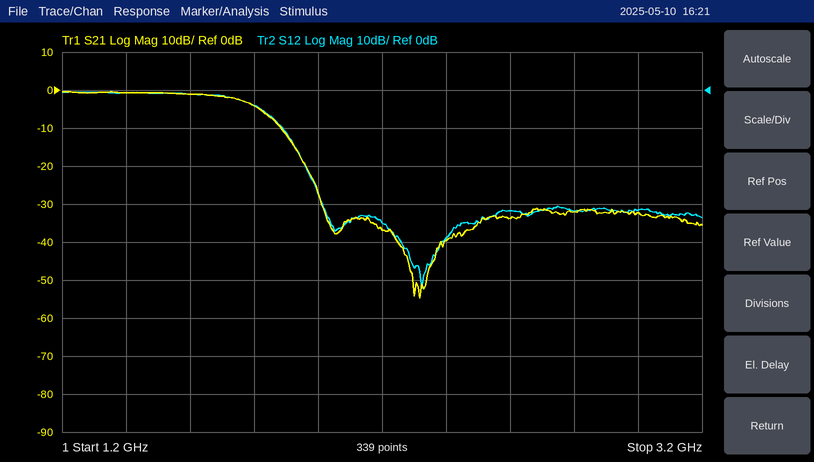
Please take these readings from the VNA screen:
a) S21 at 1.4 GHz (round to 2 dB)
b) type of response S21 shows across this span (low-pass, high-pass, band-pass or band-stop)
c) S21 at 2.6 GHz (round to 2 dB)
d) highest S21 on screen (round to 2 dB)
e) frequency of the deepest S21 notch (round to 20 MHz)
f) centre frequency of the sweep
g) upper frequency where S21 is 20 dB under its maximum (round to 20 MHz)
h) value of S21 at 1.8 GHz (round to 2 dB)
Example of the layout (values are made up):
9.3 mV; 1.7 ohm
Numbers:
0 dB; low-pass; -34 dB; 0 dB; 2.32 GHz; 2.2 GHz; 1.96 GHz; -4 dB
